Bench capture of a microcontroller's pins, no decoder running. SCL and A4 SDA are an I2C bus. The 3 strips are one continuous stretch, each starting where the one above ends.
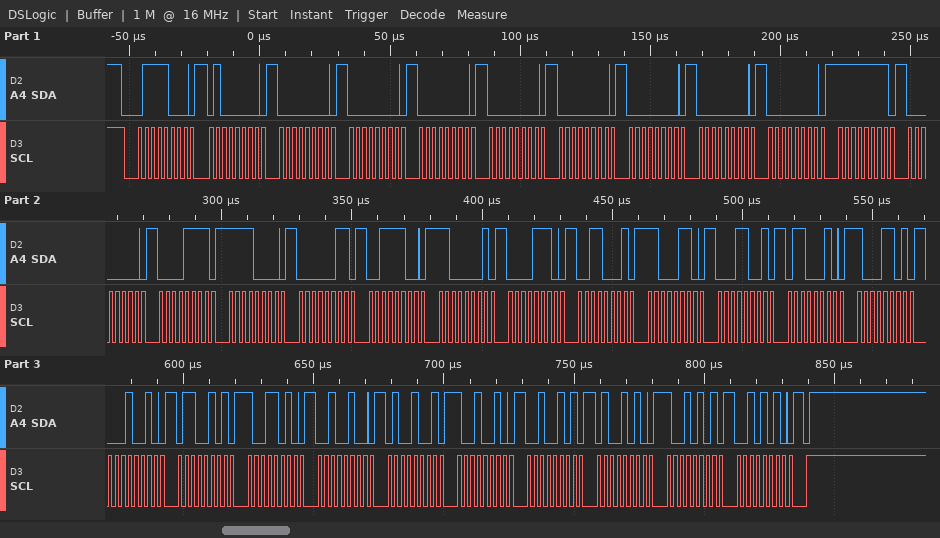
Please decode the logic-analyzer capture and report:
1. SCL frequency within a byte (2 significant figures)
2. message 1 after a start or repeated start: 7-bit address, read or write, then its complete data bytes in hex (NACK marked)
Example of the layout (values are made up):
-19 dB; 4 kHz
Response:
400 kHz; 0x3C write: 40 00 00 00 00 00 00 00 00 FF 00 0F F0 03 3C C1 0E 31 C6 19 62 8D 12 65 9A 24 49 92 25 4A 95 2A
